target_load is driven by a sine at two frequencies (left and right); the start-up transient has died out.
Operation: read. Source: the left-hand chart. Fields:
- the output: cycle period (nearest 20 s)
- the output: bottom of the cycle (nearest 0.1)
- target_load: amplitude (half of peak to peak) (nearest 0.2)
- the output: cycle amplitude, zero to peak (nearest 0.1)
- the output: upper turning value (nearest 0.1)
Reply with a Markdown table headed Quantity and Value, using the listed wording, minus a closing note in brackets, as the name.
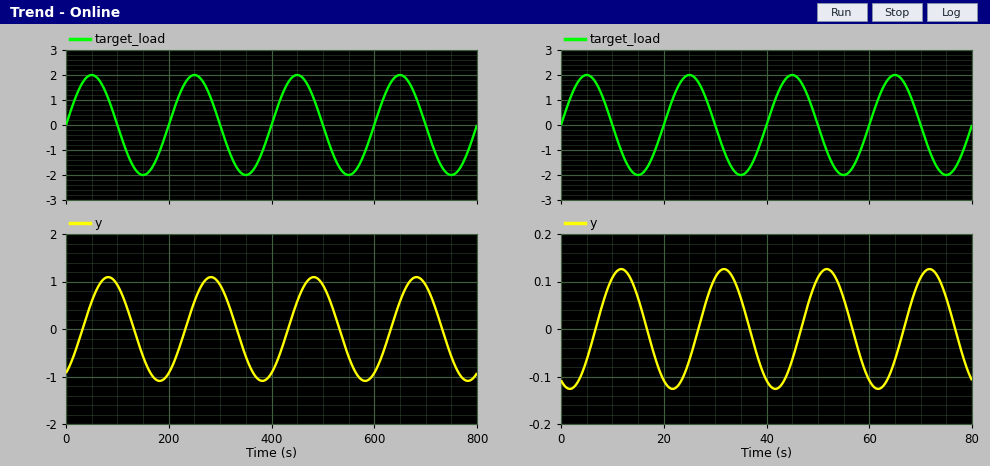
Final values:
| Quantity | Value |
|---|---|
| the output: cycle period | 200 s |
| the output: bottom of the cycle | -1.1 |
| target_load: amplitude (half of peak to peak) | 2.0 |
| the output: cycle amplitude, zero to peak | 1.1 |
| the output: upper turning value | 1.1 |
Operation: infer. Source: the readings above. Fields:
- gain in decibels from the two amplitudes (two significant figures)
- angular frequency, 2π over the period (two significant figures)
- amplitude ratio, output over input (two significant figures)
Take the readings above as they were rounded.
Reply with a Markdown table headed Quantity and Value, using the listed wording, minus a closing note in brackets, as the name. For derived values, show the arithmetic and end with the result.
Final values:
| Quantity | Value |
|---|---|
| gain in decibels from the two amplitudes | 20 log10(1.1 / 2) = -5.2 dB |
| angular frequency, 2π over the period | 2π / 200 = 0.031 rad/s |
| amplitude ratio, output over input | 1.1 / 2 = 0.55 |
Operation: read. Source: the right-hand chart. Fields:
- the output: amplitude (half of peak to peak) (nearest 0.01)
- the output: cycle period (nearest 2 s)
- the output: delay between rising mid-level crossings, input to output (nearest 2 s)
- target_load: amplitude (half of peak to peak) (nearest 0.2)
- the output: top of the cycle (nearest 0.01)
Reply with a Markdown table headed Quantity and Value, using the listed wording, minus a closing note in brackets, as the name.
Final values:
| Quantity | Value |
|---|---|
| the output: amplitude (half of peak to peak) | 0.13 |
| the output: cycle period | 20 s |
| the output: delay between rising mid-level crossings, input to output | 6 s |
| target_load: amplitude (half of peak to peak) | 2.0 |
| the output: top of the cycle | 0.13 |
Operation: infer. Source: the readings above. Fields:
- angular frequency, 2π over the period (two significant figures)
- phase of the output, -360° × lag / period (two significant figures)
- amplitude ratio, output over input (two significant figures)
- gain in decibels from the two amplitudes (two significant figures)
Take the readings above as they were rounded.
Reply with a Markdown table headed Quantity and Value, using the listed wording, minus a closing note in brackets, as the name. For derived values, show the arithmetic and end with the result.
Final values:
| Quantity | Value |
|---|---|
| angular frequency, 2π over the period | 2π / 20 = 0.31 rad/s |
| phase of the output, -360° × lag / period | -360 × 6 / 20 = -110° |
| amplitude ratio, output over input | 0.13 / 2 = 0.065 |
| gain in decibels from the two amplitudes | 20 log10(0.13 / 2) = -24 dB |
